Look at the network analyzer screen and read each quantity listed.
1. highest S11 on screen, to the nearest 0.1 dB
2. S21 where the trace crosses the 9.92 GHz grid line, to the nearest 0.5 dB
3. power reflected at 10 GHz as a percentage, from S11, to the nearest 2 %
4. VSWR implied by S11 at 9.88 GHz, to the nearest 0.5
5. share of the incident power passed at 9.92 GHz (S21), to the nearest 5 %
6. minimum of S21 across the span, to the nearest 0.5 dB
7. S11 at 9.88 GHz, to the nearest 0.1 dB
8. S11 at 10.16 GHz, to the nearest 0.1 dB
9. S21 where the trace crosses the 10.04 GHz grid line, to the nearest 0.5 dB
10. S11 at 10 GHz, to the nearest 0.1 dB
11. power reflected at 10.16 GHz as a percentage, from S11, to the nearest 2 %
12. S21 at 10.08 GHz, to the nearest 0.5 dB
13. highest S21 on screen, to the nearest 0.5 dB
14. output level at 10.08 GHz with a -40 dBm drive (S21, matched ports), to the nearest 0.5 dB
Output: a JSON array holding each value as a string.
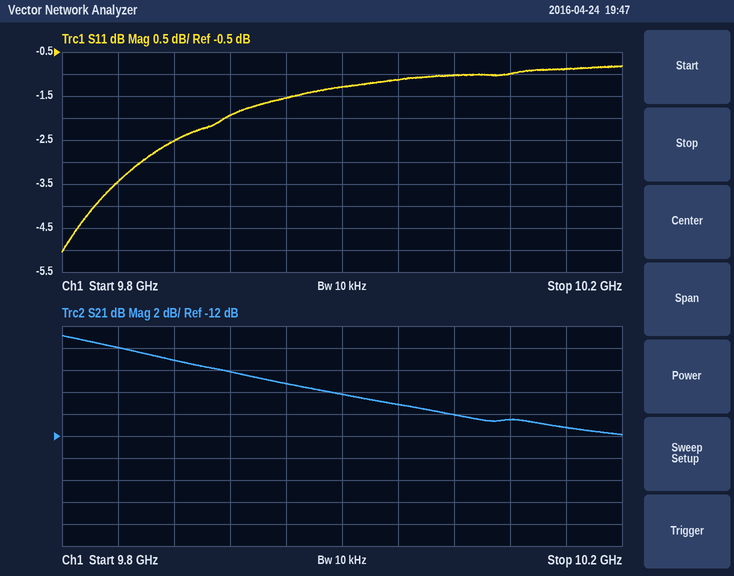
["-0.8 dB", "-6.0 dB", "74 %", "7.0", "25 %", "-12.0 dB", "-2.5 dB", "-0.9 dB", "-9.0 dB", "-1.3 dB", "82 %", "-10.0 dB", "-3.0 dB", "-50.0 dBm"]
